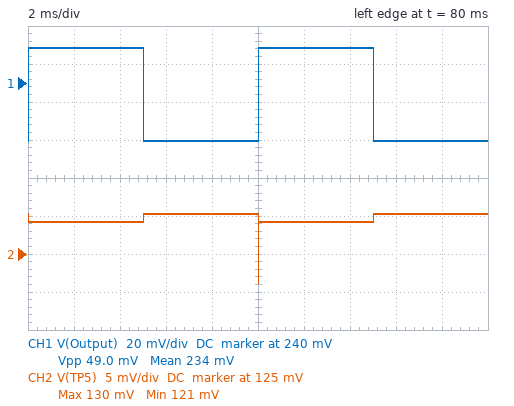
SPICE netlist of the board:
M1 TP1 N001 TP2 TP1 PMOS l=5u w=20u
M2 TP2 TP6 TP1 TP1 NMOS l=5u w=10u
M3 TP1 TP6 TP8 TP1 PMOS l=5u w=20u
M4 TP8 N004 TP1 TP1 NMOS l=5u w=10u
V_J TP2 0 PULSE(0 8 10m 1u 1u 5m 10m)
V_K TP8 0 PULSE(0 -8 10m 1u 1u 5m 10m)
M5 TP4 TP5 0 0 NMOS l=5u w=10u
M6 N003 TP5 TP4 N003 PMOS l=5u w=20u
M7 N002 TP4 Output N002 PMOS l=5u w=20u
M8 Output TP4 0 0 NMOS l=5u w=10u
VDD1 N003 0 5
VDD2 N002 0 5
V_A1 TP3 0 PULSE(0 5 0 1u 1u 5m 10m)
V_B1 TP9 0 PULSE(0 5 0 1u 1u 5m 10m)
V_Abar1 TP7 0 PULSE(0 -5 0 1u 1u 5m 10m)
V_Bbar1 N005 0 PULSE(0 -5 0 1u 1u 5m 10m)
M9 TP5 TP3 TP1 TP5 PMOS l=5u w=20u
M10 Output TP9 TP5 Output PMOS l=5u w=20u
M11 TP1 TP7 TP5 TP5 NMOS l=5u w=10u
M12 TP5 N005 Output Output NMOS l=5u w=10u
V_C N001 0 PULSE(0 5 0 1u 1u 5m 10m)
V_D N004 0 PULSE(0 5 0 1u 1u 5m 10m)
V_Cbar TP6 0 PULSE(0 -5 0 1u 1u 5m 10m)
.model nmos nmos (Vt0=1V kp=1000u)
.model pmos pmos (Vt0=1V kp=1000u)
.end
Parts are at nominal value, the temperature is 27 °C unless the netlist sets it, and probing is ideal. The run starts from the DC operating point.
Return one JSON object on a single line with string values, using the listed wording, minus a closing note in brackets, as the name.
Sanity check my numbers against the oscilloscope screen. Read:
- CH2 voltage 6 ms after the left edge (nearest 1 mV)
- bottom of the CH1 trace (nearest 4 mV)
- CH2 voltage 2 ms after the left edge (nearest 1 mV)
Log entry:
{"CH2 voltage 6 ms after the left edge": "130 mV", "bottom of the CH1 trace": "208 mV", "CH2 voltage 2 ms after the left edge": "129 mV"}
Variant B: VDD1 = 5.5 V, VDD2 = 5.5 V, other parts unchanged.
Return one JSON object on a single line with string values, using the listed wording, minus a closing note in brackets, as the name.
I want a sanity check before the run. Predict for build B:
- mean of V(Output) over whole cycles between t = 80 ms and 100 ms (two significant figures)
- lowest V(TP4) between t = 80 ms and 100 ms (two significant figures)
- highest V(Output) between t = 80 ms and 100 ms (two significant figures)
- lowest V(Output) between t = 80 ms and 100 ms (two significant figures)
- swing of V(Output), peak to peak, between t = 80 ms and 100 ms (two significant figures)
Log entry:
{"mean of V(Output) over whole cycles between t = 80 ms and 100 ms": "210 mV", "lowest V(TP4) between t = 80 ms and 100 ms": "5.5 V", "highest V(Output) between t = 80 ms and 100 ms": "230 mV", "lowest V(Output) between t = 80 ms and 100 ms": "190 mV", "swing of V(Output), peak to peak, between t = 80 ms and 100 ms": "39 mV"}
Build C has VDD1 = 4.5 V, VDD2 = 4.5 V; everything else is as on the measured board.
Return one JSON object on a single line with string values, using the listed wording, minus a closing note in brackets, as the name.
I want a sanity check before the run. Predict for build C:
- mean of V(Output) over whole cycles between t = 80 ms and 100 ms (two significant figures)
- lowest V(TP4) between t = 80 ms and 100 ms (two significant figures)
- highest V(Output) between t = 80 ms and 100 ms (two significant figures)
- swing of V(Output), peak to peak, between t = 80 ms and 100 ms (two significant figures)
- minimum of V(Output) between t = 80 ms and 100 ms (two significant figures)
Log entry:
{"mean of V(Output) over whole cycles between t = 80 ms and 100 ms": "270 mV", "lowest V(TP4) between t = 80 ms and 100 ms": "4.5 V", "highest V(Output) between t = 80 ms and 100 ms": "300 mV", "swing of V(Output), peak to peak, between t = 80 ms and 100 ms": "65 mV", "minimum of V(Output) between t = 80 ms and 100 ms": "230 mV"}
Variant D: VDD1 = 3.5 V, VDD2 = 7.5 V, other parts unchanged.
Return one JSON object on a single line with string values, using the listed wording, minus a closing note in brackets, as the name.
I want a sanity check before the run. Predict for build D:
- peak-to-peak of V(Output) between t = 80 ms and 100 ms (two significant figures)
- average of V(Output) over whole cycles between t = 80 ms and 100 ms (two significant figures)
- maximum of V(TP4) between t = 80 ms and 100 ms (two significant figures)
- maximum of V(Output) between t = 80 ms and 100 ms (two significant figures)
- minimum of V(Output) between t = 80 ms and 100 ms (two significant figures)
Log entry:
{"peak-to-peak of V(Output) between t = 80 ms and 100 ms": "720 mV", "average of V(Output) over whole cycles between t = 80 ms and 100 ms": "1.9 V", "maximum of V(TP4) between t = 80 ms and 100 ms": "3.5 V", "maximum of V(Output) between t = 80 ms and 100 ms": "2.2 V", "minimum of V(Output) between t = 80 ms and 100 ms": "1.5 V"}
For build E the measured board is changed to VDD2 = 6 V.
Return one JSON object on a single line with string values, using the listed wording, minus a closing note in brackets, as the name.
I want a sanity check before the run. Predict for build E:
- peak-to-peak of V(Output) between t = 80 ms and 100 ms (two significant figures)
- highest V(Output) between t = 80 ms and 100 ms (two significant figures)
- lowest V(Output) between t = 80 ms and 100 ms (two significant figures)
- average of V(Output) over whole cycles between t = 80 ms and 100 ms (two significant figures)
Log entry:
{"peak-to-peak of V(Output) between t = 80 ms and 100 ms": "310 mV", "highest V(Output) between t = 80 ms and 100 ms": "1.2 V", "lowest V(Output) between t = 80 ms and 100 ms": "850 mV", "average of V(Output) over whole cycles between t = 80 ms and 100 ms": "1.0 V"}
